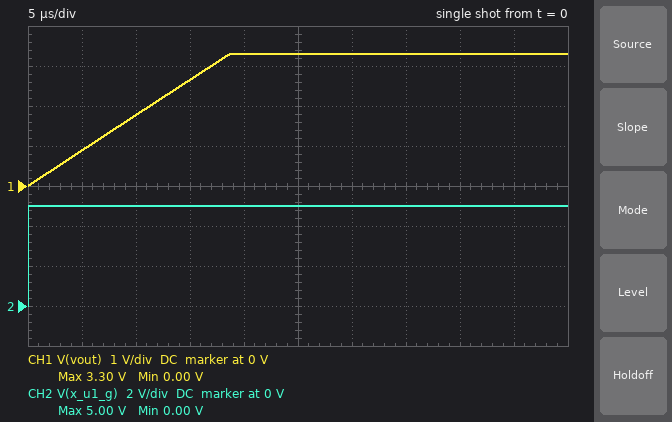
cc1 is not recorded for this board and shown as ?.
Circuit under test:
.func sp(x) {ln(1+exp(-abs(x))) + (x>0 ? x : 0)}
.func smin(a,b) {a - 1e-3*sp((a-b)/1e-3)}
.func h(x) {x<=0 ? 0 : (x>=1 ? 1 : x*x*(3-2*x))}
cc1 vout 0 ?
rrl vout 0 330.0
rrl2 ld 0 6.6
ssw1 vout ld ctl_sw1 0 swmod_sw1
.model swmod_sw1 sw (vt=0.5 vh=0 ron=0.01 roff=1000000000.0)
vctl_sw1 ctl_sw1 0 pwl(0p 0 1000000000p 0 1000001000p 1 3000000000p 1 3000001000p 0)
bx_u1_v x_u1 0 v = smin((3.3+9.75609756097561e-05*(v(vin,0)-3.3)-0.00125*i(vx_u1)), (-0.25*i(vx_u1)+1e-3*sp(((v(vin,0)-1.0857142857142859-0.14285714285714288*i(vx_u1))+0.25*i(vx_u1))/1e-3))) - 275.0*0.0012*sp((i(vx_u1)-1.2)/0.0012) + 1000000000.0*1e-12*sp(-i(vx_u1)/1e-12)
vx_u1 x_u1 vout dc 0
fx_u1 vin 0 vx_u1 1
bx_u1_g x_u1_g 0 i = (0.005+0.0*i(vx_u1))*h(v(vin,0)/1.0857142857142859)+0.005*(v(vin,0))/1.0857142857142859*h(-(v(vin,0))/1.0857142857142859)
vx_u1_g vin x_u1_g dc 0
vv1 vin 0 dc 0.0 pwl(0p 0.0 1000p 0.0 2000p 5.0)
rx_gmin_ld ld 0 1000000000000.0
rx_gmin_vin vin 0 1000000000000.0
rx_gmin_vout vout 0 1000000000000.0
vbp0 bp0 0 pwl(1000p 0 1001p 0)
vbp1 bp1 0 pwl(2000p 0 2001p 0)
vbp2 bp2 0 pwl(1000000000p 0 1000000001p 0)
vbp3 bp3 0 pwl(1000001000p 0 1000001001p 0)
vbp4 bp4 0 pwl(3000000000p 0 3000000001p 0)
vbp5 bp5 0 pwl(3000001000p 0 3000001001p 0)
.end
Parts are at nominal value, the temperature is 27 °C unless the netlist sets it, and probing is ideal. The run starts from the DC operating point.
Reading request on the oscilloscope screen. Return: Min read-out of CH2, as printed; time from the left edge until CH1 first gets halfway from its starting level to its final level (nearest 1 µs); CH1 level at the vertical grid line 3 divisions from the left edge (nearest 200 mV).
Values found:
0.00 V
9 µs
2.6 V
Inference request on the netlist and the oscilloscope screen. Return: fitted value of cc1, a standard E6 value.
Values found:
6.8 µF
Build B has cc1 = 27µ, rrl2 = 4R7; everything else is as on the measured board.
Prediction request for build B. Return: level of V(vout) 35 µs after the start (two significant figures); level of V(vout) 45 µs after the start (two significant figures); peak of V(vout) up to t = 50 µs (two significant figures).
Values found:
1.6 V
2.0 V
2.2 V
